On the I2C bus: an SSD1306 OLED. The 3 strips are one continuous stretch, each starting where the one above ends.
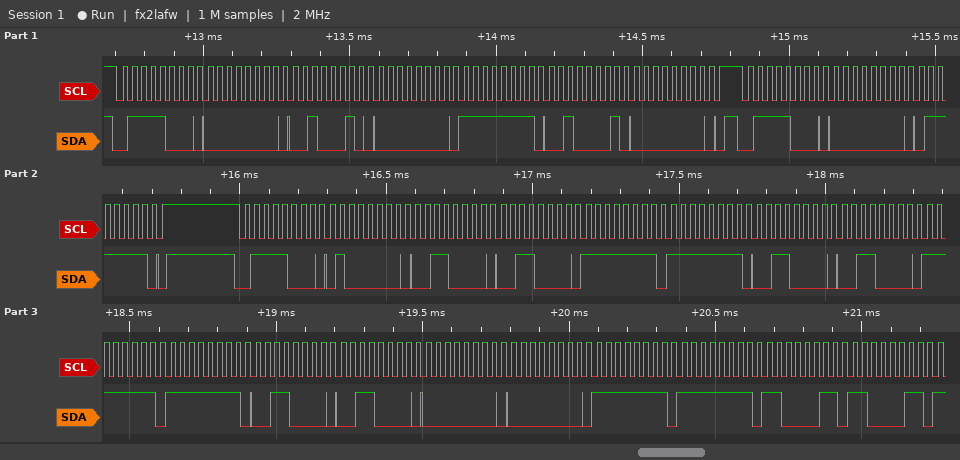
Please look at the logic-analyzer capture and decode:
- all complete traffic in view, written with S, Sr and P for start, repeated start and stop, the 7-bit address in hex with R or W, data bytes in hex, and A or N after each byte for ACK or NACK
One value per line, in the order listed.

S 3CW A 00 A 22 A 00 A FF A 21 A 00 A P S 3CW A 00 A 7F A P S 3CW A 40 A 30 A 30 A FF A FF A 30 A 30 A FF A FF A 30 A 30 A 00 A 00 A FF A FF A C3 A C3 A
